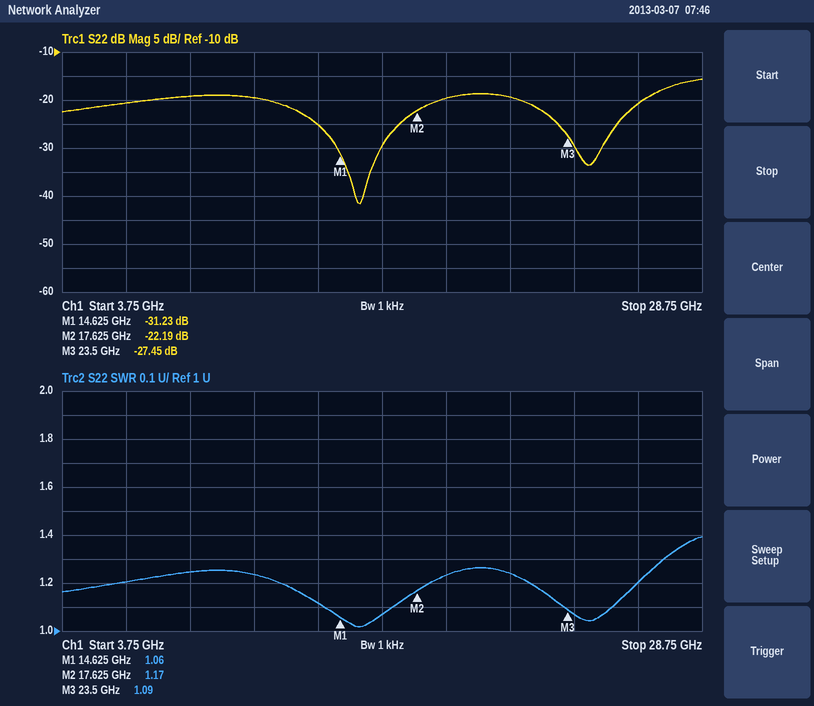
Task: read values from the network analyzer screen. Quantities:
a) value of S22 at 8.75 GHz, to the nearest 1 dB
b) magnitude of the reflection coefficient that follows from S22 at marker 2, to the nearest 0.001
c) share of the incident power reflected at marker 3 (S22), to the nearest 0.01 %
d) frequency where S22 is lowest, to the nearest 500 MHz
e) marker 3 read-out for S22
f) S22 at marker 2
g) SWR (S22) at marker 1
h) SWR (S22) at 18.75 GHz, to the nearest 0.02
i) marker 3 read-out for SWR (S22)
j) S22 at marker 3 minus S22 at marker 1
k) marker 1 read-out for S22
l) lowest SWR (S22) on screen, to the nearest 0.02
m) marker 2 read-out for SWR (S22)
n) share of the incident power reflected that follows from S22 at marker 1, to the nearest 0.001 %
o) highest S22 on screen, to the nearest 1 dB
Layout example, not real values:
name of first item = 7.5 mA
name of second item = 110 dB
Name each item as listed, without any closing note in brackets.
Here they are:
value of S22 at 8.75 GHz, to the nearest 1 dB = -19 dB
magnitude of the reflection coefficient that follows from S22 at marker 2, to the nearest 0.001 = 0.078
share of the incident power reflected at marker 3 (S22), to the nearest 0.01 % = 0.18 %
frequency where S22 is lowest, to the nearest 500 MHz = 15.5 GHz
marker 3 read-out for S22 = -27.45 dB
S22 at marker 2 = -22.19 dB
SWR (S22) at marker 1 = 1.06
SWR (S22) at 18.75 GHz, to the nearest 0.02 = 1.24
marker 3 read-out for SWR = 1.09
S22 at marker 3 minus S22 at marker 1 = 3.78 dB
marker 1 read-out for S22 = -31.23 dB
lowest SWR (S22) on screen, to the nearest 0.02 = 1.02
marker 2 read-out for SWR = 1.17
share of the incident power reflected that follows from S22 at marker 1, to the nearest 0.001 % = 0.075 %
highest S22 on screen, to the nearest 1 dB = -16 dB
